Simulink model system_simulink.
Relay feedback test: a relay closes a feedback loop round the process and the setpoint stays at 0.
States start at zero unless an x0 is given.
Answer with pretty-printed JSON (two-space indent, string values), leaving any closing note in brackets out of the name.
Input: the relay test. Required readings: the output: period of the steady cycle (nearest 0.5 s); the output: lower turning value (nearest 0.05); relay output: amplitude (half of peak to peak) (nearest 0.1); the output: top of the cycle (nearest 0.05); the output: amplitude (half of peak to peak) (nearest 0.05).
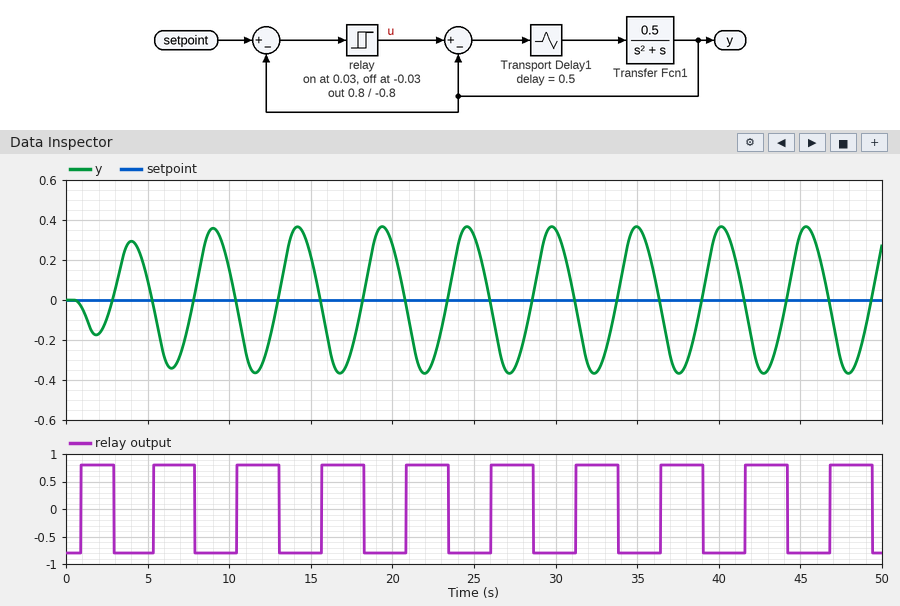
{
  "the output: period of the steady cycle": "5.0 s",
  "the output: lower turning value": "-0.35",
  "relay output: amplitude (half of peak to peak)": "0.8",
  "the output: top of the cycle": "0.35",
  "the output: amplitude (half of peak to peak)": "0.35"
}
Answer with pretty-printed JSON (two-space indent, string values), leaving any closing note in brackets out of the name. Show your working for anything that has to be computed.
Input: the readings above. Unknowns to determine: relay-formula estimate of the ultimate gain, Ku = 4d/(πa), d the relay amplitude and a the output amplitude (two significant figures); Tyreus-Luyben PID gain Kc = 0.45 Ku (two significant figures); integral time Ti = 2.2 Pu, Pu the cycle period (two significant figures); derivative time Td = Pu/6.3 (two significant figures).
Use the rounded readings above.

{
  "relay-formula estimate of the ultimate gain, Ku = 4d/(πa), d the relay amplitude and a the output amplitude": "4 × 0.8 / (π × 0.35) = 2.9",
  "Tyreus-Luyben PID gain Kc = 0.45 Ku": "0.45 × 2.9 = 1.3",
  "integral time Ti = 2.2 Pu, Pu the cycle period": "2.2 × 5 = 11 s",
  "derivative time Td = Pu/6.3": "5 / 6.3 = 0.79 s"
}
